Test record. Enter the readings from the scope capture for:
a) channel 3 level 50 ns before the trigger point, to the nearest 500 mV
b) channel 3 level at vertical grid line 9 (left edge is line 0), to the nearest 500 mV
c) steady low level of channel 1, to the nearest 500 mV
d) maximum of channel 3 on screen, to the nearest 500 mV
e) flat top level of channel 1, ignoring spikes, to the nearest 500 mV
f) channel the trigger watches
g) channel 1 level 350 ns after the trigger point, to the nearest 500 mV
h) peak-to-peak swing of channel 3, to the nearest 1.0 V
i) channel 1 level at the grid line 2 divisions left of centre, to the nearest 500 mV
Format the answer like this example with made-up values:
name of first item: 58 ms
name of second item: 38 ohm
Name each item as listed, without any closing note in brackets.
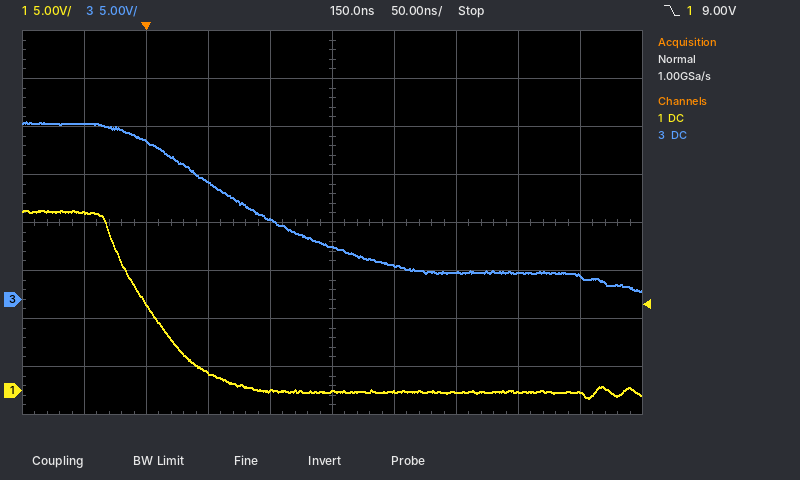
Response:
channel 3 level 50 ns before the trigger point, to the nearest 500 mV: 18.5 V
channel 3 level at vertical grid line 9 (left edge is line 0), to the nearest 500 mV: 2.5 V
steady low level of channel 1, to the nearest 500 mV: 0.0 V
maximum of channel 3 on screen, to the nearest 500 mV: 18.5 V
flat top level of channel 1, ignoring spikes, to the nearest 500 mV: 18.5 V
channel the trigger watches: channel 1
channel 1 level 350 ns after the trigger point, to the nearest 500 mV: 0.0 V
peak-to-peak swing of channel 3, to the nearest 1.0 V: 18.0 V
channel 1 level at the grid line 2 divisions left of centre, to the nearest 500 mV: 2.0 V
